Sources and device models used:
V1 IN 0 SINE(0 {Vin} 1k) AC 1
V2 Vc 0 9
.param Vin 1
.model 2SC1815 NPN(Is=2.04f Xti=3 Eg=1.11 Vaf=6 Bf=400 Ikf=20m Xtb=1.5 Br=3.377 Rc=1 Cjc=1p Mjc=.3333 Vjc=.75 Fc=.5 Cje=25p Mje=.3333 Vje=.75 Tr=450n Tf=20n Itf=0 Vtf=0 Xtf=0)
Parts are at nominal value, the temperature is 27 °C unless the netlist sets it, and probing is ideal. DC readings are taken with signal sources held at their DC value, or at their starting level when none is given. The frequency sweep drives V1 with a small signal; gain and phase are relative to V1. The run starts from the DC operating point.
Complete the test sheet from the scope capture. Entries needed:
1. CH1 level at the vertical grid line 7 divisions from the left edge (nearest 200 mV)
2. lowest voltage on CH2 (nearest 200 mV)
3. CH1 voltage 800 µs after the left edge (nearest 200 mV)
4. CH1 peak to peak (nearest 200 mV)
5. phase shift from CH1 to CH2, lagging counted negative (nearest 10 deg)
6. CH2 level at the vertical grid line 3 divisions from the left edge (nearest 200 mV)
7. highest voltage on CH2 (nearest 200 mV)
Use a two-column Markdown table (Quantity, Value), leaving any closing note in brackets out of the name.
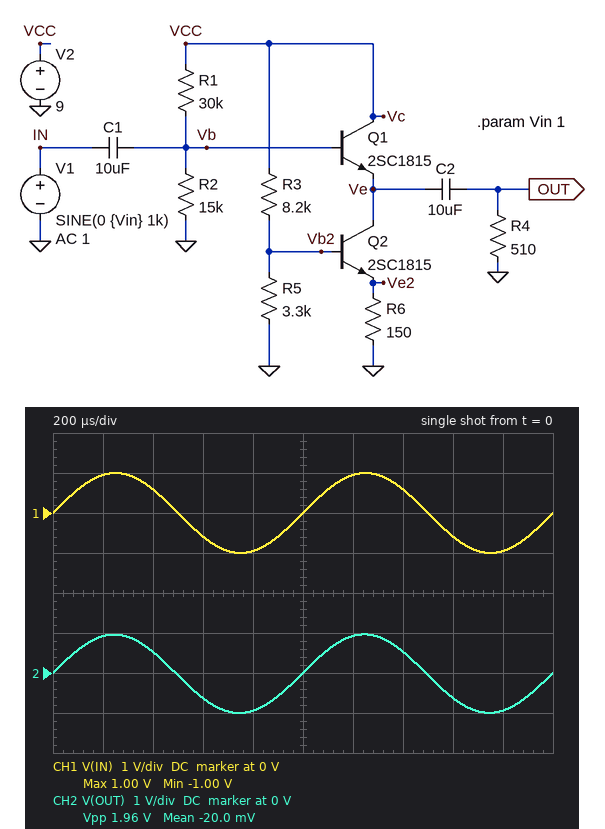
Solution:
| Quantity | Value |
|---|---|
| CH1 level at the vertical grid line 7 divisions from the left edge | 600 mV |
| lowest voltage on CH2 | -1.0 V |
| CH1 voltage 800 µs after the left edge | -1.0 V |
| CH1 peak to peak | 2.0 V |
| phase shift from CH1 to CH2, lagging counted negative | 0 deg |
| CH2 level at the vertical grid line 3 divisions from the left edge | -600 mV |
| highest voltage on CH2 | 1.0 V |
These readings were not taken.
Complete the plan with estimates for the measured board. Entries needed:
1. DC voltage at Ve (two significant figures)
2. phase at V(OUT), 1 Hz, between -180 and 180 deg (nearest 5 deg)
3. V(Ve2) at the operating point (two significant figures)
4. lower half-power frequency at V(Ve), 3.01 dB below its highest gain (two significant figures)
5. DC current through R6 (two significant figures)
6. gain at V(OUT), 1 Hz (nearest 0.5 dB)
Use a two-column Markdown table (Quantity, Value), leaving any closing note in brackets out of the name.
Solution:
| Quantity | Value |
|---|---|
| DC voltage at Ve | 2.1 V |
| phase at V(OUT), 1 Hz, between -180 and 180 deg | 145 deg |
| V(Ve2) at the operating point | 1.7 V |
| lower half-power frequency at V(Ve), 3.01 dB below its highest gain | 1.6 Hz |
| DC current through R6 | 11 mA |
| gain at V(OUT), 1 Hz | -35.5 dB |
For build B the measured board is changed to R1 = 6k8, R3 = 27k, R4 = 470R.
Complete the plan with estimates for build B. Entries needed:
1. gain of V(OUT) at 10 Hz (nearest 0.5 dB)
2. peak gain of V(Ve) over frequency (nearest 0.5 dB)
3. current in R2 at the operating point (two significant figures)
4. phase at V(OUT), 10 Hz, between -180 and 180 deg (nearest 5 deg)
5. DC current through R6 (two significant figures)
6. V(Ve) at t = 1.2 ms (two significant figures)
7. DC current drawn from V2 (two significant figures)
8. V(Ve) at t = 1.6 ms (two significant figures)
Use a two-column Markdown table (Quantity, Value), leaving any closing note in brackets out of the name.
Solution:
| Quantity | Value |
|---|---|
| gain of V(OUT) at 10 Hz | -11.5 dB |
| peak gain of V(Ve) over frequency | 0 dB |
| current in R2 at the operating point | 410 µA |
| phase at V(OUT), 10 Hz, between -180 and 180 deg | 90 deg |
| DC current through R6 | 1.8 mA |
| V(Ve) at t = 1.2 ms | 6.4 V |
| DC current drawn from V2 | 2.5 mA |
| V(Ve) at t = 1.6 ms | 4.9 V |
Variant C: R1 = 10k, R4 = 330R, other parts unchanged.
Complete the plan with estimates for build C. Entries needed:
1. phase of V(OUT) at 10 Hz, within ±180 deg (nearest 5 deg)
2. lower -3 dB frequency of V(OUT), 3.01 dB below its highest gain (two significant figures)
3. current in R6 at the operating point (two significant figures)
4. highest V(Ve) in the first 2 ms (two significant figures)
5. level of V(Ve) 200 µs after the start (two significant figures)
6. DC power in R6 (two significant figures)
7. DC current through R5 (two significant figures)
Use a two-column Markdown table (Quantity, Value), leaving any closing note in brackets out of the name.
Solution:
| Quantity | Value |
|---|---|
| phase of V(OUT) at 10 Hz, within ±180 deg | 95 deg |
| lower -3 dB frequency of V(OUT), 3.01 dB below its highest gain | 48 Hz |
| current in R6 at the operating point | 12 mA |
| highest V(Ve) in the first 2 ms | 5.5 V |
| level of V(Ve) 200 µs after the start | 5.4 V |
| DC power in R6 | 20 mW |
| DC current through R5 | 760 µA |
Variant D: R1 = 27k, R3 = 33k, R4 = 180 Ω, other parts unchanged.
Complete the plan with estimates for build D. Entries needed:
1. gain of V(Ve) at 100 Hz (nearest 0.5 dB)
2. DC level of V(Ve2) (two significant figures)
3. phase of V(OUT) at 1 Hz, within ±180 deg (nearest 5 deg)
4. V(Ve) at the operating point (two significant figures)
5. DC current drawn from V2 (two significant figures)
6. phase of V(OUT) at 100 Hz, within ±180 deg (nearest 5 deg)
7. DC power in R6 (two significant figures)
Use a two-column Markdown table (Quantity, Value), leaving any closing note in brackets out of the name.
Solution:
| Quantity | Value |
|---|---|
| gain of V(Ve) at 100 Hz | -1.0 dB |
| DC level of V(Ve2) | 130 mV |
| phase of V(OUT) at 1 Hz, within ±180 deg | 150 deg |
| V(Ve) at the operating point | 2.5 V |
| DC current drawn from V2 | 1.3 mA |
| phase of V(OUT) at 100 Hz, within ±180 deg | 40 deg |
| DC power in R6 | 110 µW |
